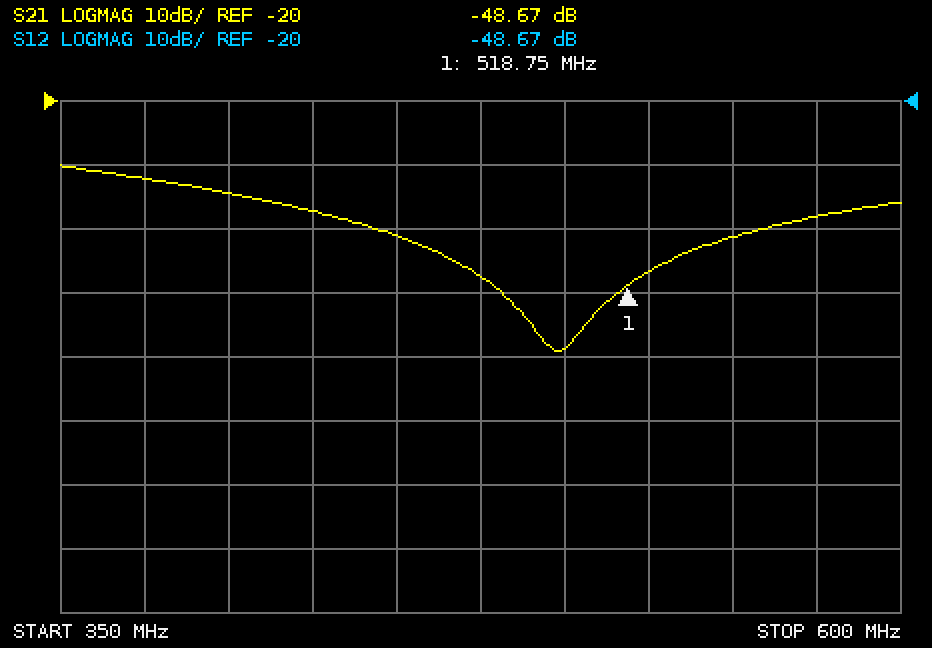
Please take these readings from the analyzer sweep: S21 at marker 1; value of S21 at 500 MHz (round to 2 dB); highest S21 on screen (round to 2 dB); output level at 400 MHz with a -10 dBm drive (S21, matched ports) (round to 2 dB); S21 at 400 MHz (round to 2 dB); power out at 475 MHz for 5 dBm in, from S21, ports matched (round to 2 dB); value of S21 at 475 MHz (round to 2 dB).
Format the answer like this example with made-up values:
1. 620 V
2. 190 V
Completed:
1. -48.67 dB
2. -58 dB
3. -30 dB
4. -44 dBm
5. -34 dB
6. -42 dBm
7. -48 dB
